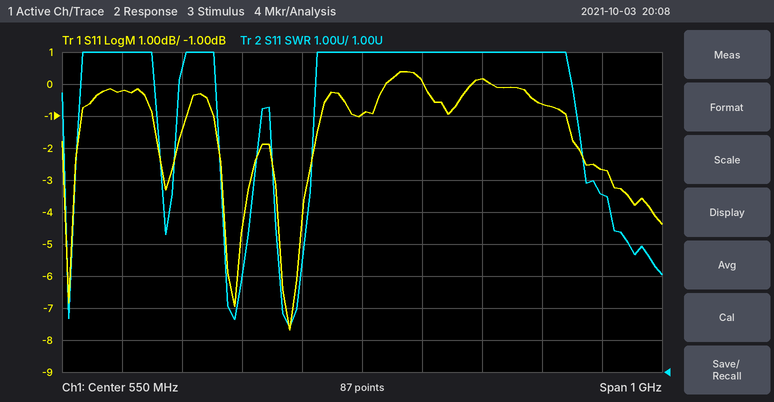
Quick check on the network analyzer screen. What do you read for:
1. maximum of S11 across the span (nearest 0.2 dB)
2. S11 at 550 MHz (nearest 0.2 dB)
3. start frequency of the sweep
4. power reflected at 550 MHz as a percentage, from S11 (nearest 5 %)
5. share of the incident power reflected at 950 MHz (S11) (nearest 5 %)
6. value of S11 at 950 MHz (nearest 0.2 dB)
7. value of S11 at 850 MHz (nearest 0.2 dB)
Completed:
0.4 dB
-1.0 dB
50 MHz
80 %
55 %
-2.6 dB
-0.6 dB
